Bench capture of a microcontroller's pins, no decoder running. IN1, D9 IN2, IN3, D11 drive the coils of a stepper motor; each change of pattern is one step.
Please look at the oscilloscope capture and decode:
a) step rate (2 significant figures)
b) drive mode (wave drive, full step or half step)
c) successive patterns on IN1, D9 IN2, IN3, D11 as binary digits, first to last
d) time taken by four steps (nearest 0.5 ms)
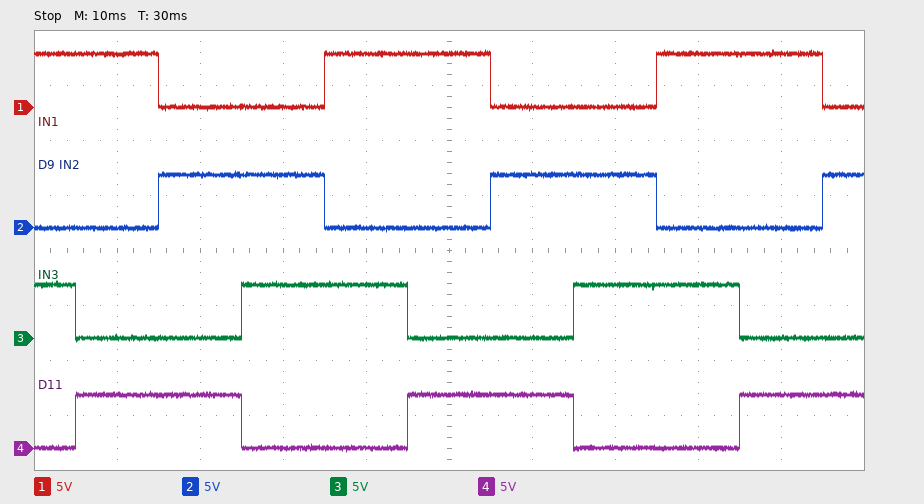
100 steps/s
full step
1010 1001 0101 0110 1010 1001 0101 0110 1010 1001 0101
40.0 ms
